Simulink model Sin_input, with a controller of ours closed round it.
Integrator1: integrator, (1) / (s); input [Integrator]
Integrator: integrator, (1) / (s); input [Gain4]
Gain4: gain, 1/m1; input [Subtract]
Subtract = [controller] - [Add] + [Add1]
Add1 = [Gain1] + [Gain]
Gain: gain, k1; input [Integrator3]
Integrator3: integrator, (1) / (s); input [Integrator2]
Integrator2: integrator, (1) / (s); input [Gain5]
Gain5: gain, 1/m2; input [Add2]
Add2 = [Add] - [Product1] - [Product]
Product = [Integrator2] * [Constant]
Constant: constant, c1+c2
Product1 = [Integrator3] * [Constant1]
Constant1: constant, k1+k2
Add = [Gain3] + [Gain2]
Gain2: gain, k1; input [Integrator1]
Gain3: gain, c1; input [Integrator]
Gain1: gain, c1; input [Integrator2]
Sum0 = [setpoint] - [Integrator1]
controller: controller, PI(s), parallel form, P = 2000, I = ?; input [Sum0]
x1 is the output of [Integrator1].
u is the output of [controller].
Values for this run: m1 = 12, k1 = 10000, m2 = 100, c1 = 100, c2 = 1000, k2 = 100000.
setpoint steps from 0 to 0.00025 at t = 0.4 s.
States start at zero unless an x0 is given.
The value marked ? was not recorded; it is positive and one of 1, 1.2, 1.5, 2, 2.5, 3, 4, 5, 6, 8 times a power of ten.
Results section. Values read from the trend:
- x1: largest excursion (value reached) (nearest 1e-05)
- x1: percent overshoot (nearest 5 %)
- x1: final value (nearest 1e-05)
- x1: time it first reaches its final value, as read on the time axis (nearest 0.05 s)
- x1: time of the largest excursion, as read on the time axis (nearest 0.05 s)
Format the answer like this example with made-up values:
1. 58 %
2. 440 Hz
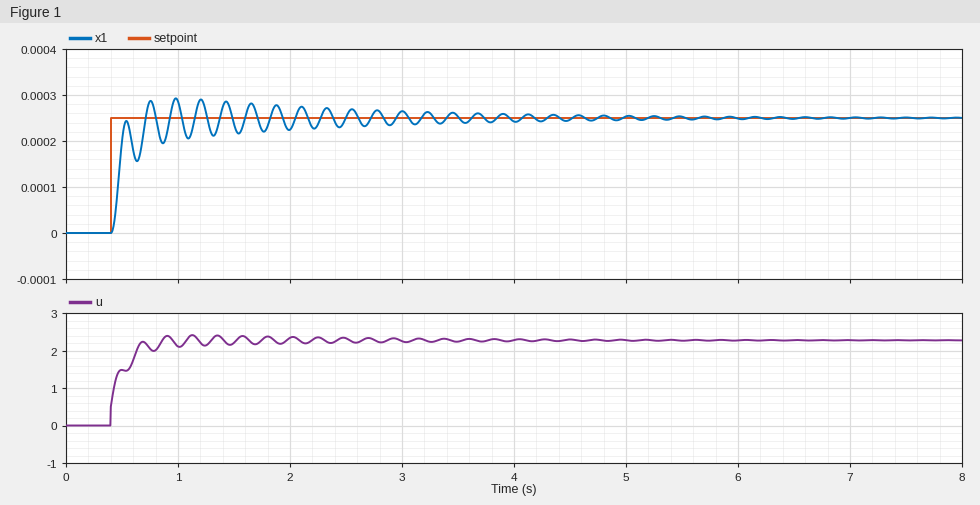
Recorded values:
1. 0.00029
2. 15 %
3. 0.00025
4. 0.70 s
5. 1.00 s
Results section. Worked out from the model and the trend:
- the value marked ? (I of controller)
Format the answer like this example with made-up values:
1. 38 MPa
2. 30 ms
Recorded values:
1. 80000
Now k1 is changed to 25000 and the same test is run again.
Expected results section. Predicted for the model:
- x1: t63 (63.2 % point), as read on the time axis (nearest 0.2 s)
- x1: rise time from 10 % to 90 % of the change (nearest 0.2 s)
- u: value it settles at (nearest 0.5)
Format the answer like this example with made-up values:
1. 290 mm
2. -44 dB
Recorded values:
1. 0.6 s
2. 0.6 s
3. 5.0
